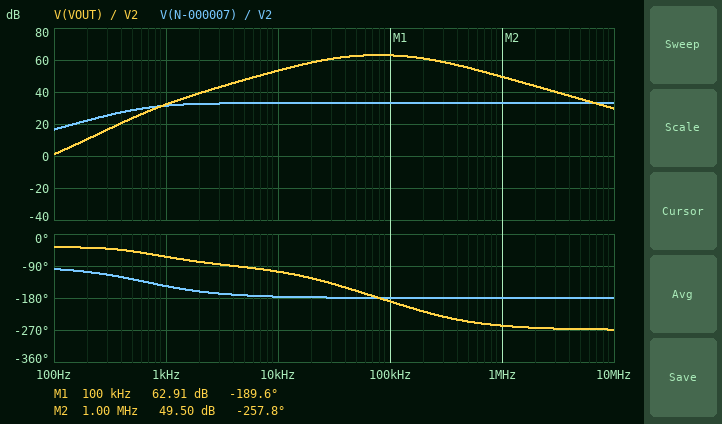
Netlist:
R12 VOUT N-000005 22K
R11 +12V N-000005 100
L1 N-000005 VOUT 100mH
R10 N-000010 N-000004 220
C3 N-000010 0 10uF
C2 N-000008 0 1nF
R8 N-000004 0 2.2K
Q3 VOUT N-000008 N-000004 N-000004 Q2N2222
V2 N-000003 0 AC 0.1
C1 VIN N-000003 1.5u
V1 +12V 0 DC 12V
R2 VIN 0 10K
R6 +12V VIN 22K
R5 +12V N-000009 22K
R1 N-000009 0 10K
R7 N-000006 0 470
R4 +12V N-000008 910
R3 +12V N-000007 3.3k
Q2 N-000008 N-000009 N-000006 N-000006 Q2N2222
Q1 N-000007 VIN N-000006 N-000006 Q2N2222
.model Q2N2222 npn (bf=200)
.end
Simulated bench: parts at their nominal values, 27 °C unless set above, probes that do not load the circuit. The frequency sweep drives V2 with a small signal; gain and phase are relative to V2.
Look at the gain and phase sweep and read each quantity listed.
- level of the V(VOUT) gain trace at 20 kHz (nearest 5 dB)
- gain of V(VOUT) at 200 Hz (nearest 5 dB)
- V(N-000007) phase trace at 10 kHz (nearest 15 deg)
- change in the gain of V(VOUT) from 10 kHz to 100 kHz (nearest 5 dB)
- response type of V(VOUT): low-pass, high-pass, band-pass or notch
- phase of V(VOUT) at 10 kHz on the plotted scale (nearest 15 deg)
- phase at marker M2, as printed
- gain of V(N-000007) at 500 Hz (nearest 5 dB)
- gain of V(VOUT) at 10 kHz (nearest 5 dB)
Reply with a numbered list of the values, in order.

1. 60 dB
2. 10 dB
3. -180 deg
4. 10 dB
5. band-pass
6. -105 deg
7. -257.8 deg
8. 30 dB
9. 55 dB
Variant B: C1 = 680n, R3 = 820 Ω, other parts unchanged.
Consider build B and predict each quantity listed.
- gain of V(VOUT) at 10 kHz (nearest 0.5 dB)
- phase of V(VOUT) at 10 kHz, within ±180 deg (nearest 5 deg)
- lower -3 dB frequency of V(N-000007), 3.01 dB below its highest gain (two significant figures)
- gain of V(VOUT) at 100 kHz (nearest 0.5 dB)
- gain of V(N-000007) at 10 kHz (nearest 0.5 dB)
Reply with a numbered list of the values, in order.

1. 54.0 dB
2. -110 deg
3. 58 Hz
4. 63.5 dB
5. 24.5 dB
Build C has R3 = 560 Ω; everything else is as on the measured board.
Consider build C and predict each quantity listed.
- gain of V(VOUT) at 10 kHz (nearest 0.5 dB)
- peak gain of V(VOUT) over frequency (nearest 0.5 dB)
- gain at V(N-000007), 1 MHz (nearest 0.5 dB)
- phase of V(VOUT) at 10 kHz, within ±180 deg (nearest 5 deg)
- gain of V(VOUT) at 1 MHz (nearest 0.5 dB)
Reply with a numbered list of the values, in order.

1. 54.0 dB
2. 63.5 dB
3. 21.5 dB
4. -110 deg
5. 50.0 dB
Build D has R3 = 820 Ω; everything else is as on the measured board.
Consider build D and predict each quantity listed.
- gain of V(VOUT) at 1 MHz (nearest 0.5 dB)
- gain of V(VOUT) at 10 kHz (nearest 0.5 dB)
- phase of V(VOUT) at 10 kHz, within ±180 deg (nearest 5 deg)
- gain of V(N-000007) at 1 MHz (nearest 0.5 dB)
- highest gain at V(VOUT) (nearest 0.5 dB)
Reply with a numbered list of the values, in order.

1. 50.0 dB
2. 54.0 dB
3. -110 deg
4. 24.5 dB
5. 63.5 dB
